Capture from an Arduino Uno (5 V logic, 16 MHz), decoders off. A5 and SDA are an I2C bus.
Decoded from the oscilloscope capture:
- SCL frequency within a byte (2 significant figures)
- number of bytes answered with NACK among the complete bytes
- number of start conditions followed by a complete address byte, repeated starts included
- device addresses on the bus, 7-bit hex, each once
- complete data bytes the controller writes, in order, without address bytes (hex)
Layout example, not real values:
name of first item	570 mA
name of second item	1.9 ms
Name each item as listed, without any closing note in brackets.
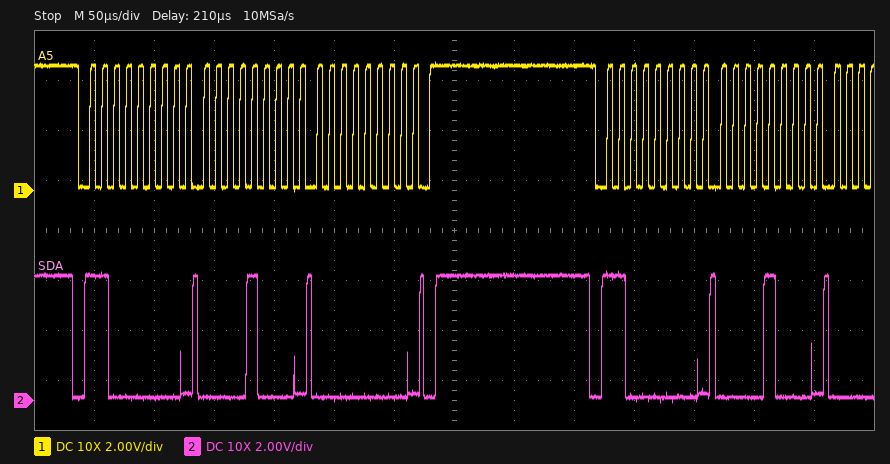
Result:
SCL frequency within a byte	100 kHz
number of bytes answered with NACK among the complete bytes	0
number of start conditions followed by a complete address byte, repeated starts included	2
device addresses on the bus, 7-bit hex, each once	0x60
complete data bytes the controller writes, in order, without address bytes	08 00 08
